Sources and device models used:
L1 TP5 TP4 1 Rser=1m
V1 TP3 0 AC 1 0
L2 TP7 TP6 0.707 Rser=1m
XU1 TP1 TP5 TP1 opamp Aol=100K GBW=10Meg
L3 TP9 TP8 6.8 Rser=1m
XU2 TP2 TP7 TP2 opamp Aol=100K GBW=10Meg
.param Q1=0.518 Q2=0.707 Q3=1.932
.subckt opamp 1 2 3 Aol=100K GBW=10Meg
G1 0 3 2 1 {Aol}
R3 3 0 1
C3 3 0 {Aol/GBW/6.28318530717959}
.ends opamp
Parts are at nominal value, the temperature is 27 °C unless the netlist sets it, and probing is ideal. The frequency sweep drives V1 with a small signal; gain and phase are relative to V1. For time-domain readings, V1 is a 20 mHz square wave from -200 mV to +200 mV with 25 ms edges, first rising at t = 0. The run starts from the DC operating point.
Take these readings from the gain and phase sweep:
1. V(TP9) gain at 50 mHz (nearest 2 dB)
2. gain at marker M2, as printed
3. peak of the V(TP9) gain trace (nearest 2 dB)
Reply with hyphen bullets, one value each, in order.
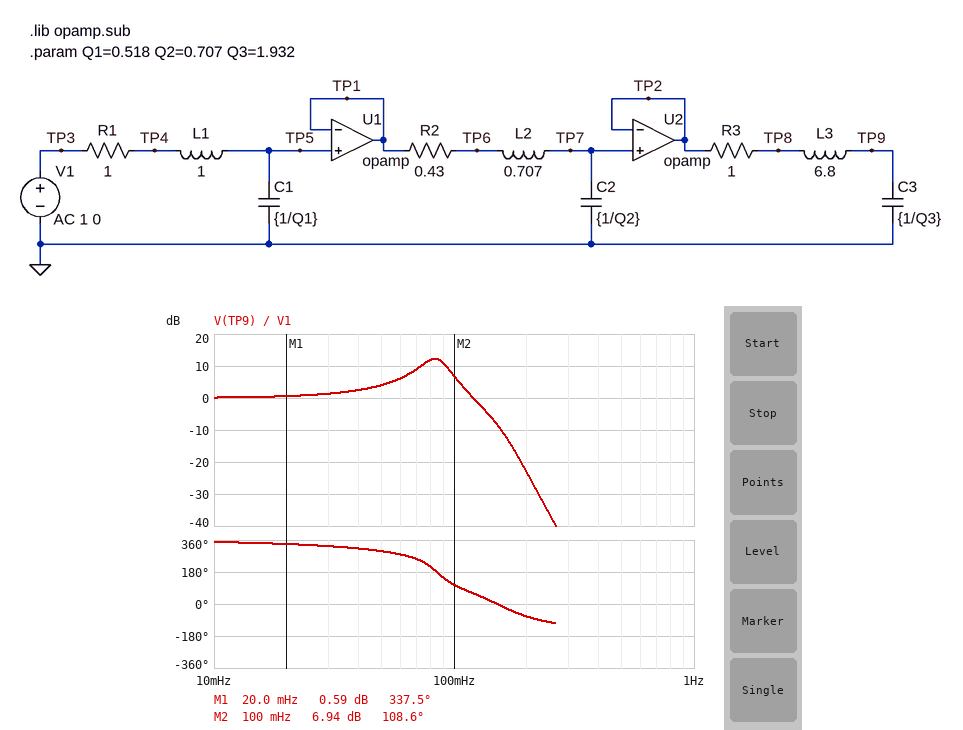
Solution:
- 4 dB
- 6.94 dB
- 12 dB
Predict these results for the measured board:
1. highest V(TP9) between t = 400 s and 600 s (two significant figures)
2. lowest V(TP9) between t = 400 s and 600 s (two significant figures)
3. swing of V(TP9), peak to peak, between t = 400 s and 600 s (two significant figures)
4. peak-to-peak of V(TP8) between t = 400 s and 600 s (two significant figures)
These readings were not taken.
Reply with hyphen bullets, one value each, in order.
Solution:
- 470 mV
- -470 mV
- 940 mV
- 530 mV
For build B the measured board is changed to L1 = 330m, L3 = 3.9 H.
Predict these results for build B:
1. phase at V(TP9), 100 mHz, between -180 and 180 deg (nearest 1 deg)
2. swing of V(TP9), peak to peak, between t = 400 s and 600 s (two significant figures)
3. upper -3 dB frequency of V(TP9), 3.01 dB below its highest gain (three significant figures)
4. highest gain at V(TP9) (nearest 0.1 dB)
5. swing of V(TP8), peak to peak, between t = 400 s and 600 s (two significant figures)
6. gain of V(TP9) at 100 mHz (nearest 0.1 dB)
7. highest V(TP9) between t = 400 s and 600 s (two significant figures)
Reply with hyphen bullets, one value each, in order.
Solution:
- -149 deg
- 840 mV
- 128 mHz
- 8.8 dB
- 510 mV
- 8.1 dB
- 420 mV
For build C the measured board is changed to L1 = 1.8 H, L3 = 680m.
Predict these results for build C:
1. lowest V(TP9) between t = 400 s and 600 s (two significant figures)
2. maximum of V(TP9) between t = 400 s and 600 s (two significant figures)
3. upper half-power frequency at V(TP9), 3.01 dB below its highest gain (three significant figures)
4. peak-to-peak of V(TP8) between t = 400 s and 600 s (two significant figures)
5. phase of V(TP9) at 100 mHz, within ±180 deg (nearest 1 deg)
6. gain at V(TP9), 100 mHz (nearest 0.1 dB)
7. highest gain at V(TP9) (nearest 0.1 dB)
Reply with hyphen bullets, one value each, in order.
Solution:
- -320 mV
- 320 mV
- 127 mHz
- 610 mV
- -160 deg
- 1.5 dB
- 2.6 dB
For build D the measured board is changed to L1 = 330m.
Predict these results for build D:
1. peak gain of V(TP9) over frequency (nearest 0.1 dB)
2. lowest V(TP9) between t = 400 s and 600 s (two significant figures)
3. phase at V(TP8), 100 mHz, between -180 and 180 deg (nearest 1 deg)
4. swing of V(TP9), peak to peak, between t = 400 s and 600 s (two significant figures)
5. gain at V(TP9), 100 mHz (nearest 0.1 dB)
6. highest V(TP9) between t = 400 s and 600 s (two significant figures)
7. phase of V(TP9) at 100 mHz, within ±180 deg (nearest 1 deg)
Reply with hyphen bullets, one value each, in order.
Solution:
- 11.0 dB
- -420 mV
- -51 deg
- 850 mV
- 5.7 dB
- 420 mV
- 129 deg
